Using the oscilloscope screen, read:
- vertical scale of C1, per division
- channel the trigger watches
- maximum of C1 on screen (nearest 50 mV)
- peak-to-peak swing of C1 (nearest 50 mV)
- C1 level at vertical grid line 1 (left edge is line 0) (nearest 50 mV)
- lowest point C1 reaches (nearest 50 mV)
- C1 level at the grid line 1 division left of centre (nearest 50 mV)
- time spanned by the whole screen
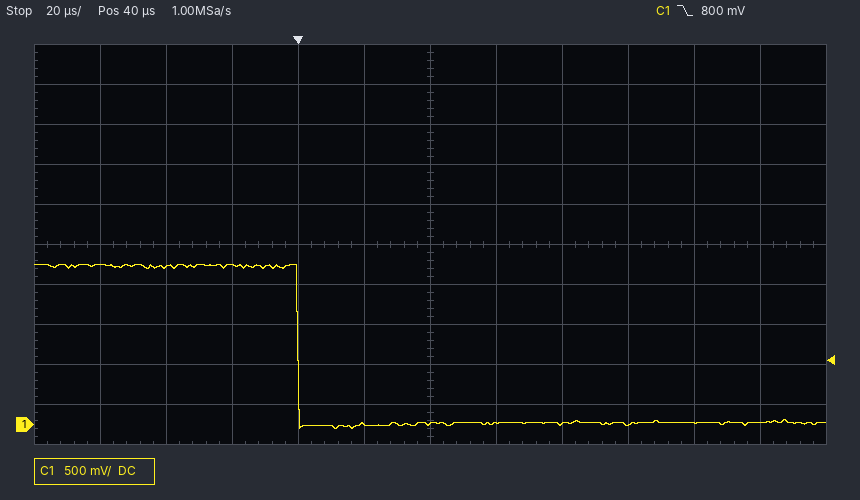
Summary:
500 mV
C1
2.00 V
2.05 V
2.00 V
-50 mV
0 mV
240 µs
